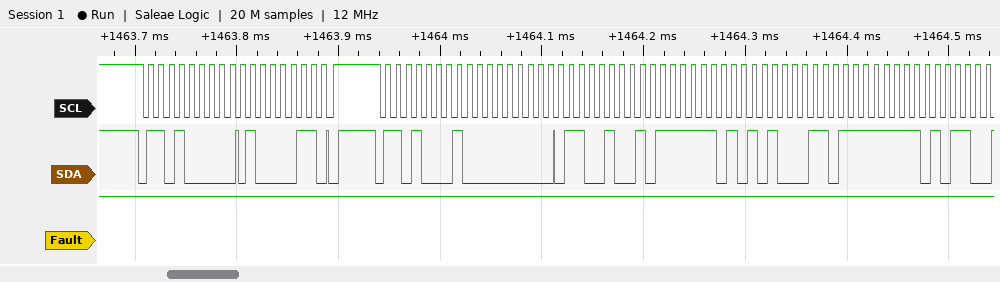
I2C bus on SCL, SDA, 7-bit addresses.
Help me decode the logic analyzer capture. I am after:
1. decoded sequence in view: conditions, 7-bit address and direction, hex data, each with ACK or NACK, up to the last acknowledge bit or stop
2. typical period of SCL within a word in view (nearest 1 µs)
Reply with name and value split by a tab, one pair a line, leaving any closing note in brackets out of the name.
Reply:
decoded sequence in view: conditions, 7-bit address and direction, hex data, each with ACK or NACK, up to the last acknowledge bit or stop	start, address 68 write ACK, 43 ACK, stop, start, address 68 read ACK, 00 ACK, C9 ACK, FD ACK, A3 ACK, FF ACK
typical period of SCL within a word in view	10 µs
